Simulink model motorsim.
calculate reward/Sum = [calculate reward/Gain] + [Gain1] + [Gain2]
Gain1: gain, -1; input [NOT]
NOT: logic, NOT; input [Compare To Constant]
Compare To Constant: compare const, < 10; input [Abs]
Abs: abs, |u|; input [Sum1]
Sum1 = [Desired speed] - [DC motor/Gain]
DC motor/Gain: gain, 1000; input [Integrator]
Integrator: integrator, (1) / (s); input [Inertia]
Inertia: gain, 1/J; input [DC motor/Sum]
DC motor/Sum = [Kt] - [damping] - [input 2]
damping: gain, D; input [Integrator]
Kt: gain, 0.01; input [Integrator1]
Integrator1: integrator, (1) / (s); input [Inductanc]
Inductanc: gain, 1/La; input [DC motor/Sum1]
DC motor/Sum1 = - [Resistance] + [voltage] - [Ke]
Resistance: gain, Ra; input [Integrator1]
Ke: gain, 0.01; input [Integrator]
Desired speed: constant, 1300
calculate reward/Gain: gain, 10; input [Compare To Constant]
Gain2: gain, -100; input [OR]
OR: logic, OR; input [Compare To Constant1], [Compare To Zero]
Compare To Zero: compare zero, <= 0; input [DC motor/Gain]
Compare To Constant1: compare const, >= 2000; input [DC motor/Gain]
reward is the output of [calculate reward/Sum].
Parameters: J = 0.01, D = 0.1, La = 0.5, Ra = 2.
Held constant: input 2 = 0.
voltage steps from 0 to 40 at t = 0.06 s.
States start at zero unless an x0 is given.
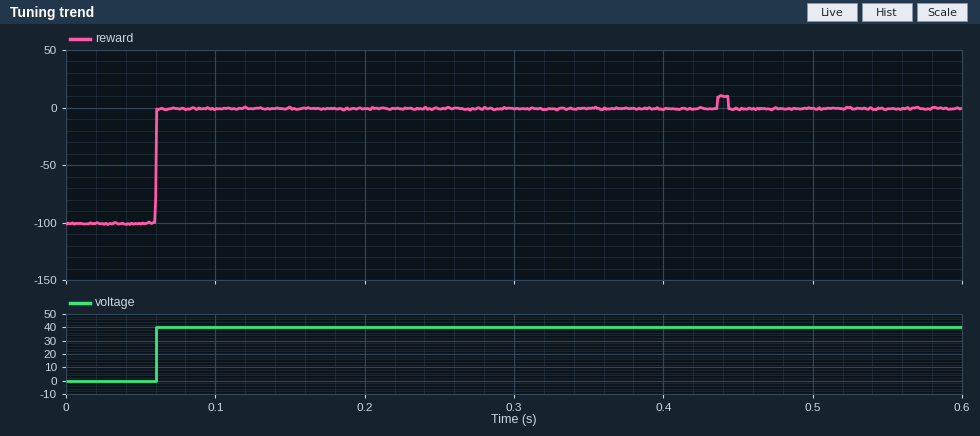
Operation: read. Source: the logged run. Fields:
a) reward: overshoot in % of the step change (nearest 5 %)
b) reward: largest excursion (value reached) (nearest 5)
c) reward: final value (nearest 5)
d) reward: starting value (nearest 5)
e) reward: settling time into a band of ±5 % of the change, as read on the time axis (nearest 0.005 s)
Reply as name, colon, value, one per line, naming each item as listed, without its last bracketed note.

reward: overshoot in % of the step change: 10 %
reward: largest excursion (value reached): 10
reward: final value: 0
reward: starting value: -100
reward: settling time into a band of ±5 % of the change, as read on the time axis: 0.445 s
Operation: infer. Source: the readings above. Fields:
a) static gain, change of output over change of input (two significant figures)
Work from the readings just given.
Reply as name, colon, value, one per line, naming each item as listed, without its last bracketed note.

static gain, change of output over change of input: 2.5
